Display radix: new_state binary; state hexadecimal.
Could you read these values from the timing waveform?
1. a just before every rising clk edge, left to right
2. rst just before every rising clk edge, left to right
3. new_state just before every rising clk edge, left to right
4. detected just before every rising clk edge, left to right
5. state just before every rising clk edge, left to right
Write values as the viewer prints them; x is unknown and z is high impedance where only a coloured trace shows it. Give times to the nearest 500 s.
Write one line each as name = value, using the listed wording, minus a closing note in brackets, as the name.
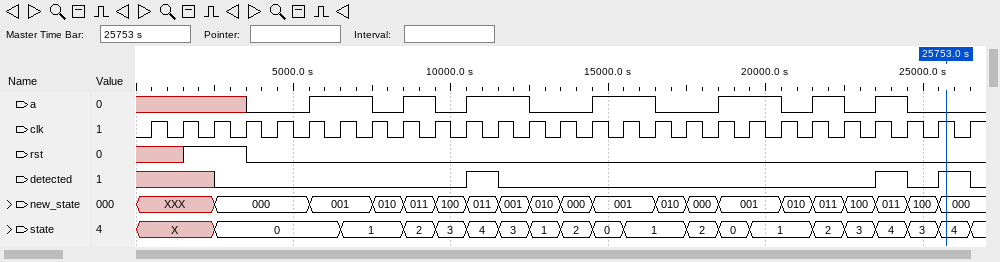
a just before every rising clk edge, left to right = x x x x 0 0 1 1 0 1 0 1 1 0 0 1 1 0 0 1 1 0 1 0 1 0 0
rst just before every rising clk edge, left to right = x x 1 1 0 0 0 0 0 0 0 0 0 0 0 0 0 0 0 0 0 0 0 0 0 0 0
new_state just before every rising clk edge, left to right = XXX, XXX, XXX, 000, 000, 000, 001, 001, 010, 011, 100, 011, 001, 010, 000, 001, 001, 010, 000, 001, 001, 010, 011, 100, 011, 100, 000
detected just before every rising clk edge, left to right = x x x 0 0 0 0 0 0 0 0 1 0 0 0 0 0 0 0 0 0 0 0 0 1 0 1
state just before every rising clk edge, left to right = X, X, X, 0, 0, 0, 0, 1, 1, 2, 3, 4, 3, 1, 2, 0, 1, 1, 2, 0, 1, 1, 2, 3, 4, 3, 4
